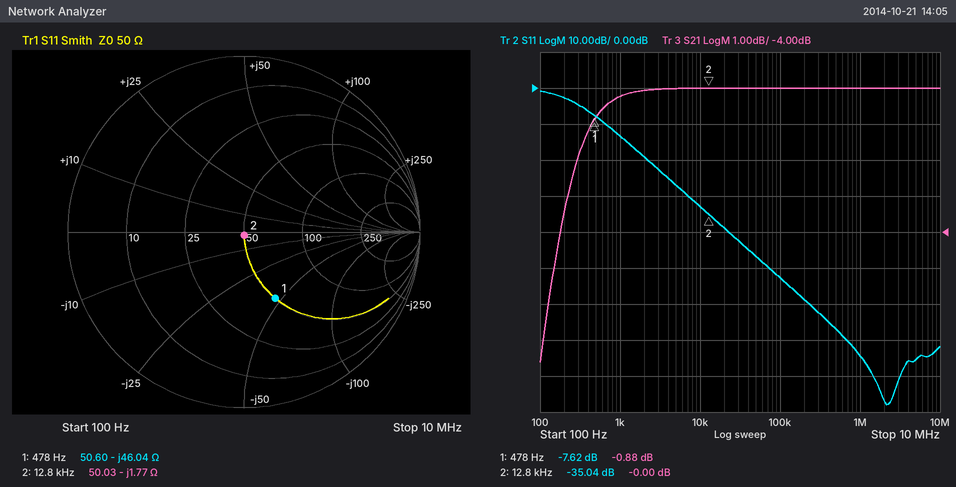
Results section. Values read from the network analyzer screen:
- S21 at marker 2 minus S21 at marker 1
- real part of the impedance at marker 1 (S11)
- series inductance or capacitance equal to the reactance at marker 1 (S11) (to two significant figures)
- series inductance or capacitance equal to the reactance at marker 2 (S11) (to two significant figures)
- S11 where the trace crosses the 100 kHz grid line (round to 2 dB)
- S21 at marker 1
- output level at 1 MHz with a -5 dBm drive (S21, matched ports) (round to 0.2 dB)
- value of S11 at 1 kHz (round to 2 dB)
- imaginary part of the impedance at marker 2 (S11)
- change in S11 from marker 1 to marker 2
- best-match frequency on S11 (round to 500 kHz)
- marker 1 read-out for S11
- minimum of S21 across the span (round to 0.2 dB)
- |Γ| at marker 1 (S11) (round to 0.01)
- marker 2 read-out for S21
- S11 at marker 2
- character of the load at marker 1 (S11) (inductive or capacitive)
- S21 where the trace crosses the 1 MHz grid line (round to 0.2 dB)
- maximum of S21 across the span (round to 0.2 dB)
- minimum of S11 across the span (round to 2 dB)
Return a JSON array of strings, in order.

["0.88 dB", "50.60 Ω", "7.2 µF", "7.0 µF", "-52 dB", "-0.88 dB", "-5.0 dBm", "-14 dB", "-1.77 Ω", "-27.42 dB", "2.0 MHz", "-7.62 dB", "-7.6 dB", "0.42", "-0.00 dB", "-35.04 dB", "capacitive", "0.0 dB", "0.0 dB", "-88 dB"]
